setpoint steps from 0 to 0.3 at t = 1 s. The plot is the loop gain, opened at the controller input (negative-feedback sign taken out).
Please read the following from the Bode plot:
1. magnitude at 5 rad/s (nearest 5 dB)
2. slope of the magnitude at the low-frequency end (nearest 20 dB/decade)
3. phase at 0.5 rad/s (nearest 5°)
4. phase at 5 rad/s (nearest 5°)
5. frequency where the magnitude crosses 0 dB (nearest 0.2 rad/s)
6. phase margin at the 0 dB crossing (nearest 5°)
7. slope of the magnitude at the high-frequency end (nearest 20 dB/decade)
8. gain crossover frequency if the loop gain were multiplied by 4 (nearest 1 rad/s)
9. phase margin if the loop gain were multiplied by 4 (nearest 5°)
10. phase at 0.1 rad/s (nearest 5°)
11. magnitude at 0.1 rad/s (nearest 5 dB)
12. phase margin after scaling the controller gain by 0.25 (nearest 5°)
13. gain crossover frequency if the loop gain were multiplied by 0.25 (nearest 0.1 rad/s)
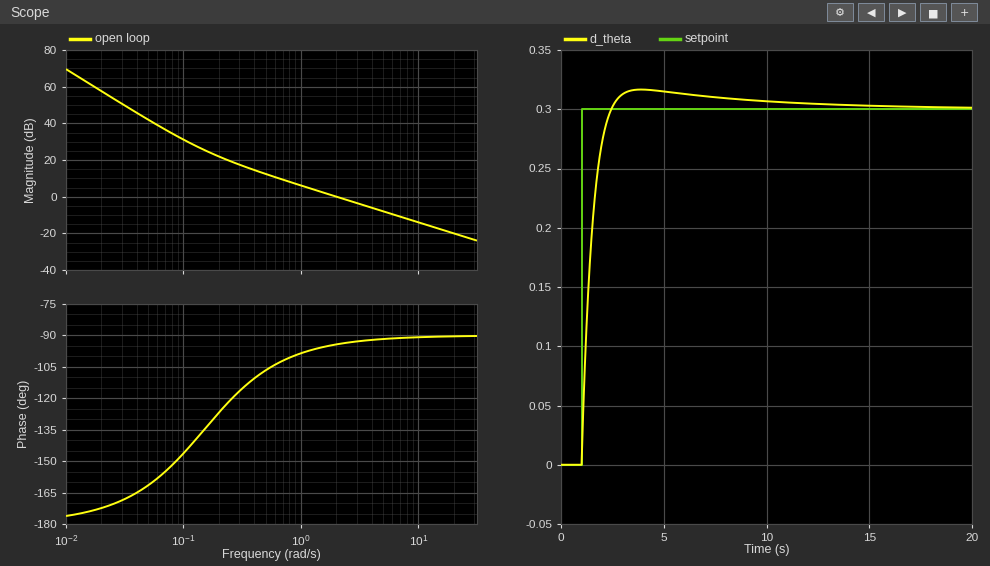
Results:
-10 dB
-40 dB/decade
-105°
-90°
2.0 rad/s
85°
-20 dB/decade
8 rad/s
90°
-145°
30 dB
75°
0.5 rad/s
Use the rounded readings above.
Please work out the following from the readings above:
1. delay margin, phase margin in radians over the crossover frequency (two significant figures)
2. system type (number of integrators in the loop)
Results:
0.74 s
2
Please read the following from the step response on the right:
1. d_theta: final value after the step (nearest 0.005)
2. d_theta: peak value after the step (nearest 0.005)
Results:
0.300
0.315
